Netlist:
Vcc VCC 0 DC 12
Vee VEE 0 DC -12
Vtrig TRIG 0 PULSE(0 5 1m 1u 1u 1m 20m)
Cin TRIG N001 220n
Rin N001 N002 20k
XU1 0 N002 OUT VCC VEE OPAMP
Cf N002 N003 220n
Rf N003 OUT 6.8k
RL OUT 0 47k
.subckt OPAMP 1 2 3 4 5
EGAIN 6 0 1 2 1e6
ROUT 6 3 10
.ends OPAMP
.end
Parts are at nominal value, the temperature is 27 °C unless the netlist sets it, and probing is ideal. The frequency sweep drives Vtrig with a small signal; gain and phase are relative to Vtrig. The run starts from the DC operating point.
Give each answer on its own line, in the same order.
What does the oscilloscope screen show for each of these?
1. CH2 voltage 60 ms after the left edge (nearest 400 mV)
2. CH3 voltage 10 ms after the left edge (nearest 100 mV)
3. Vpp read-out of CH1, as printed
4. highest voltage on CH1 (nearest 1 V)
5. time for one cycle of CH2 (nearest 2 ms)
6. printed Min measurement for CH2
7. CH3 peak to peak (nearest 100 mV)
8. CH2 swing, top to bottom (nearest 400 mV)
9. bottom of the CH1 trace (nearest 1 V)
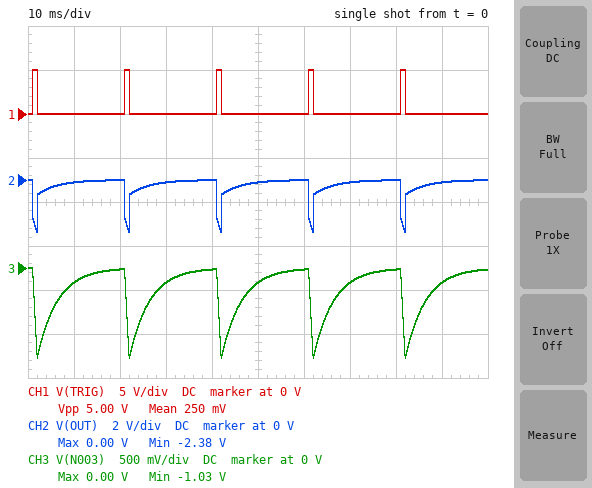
0 V
-200 mV
5.00 V
5 V
20 ms
-2.38 V
1.0 V
2.4 V
0 V
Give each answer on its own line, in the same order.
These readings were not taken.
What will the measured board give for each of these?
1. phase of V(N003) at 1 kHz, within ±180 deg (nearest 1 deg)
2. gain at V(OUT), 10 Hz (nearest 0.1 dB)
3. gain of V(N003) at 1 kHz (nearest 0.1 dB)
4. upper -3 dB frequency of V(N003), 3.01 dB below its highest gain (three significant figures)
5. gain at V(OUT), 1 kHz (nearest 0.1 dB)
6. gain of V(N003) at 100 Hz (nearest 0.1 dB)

92 deg
-0.3 dB
-28.8 dB
36.2 Hz
-9.3 dB
-9.4 dB
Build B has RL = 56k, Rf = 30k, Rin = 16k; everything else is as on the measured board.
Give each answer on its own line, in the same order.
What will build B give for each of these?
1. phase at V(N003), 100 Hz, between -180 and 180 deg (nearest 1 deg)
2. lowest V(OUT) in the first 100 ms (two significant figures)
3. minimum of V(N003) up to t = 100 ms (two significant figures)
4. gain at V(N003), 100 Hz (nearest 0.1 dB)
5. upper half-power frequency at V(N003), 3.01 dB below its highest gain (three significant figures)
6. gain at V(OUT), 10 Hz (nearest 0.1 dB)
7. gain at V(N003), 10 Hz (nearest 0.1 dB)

114 deg
-9.4 V
-1.2 V
-7.7 dB
45.2 Hz
0.5 dB
-0.2 dB
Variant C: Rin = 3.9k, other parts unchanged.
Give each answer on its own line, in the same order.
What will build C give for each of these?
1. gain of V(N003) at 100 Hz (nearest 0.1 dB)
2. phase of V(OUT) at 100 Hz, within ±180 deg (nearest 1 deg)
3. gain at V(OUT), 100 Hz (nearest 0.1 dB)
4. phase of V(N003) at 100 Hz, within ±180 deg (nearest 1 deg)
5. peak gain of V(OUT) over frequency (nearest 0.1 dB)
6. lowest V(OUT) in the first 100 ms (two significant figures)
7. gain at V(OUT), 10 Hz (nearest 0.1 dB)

-1.1 dB
-165 deg
1.6 dB
152 deg
4.8 dB
-8.7 V
0 dB
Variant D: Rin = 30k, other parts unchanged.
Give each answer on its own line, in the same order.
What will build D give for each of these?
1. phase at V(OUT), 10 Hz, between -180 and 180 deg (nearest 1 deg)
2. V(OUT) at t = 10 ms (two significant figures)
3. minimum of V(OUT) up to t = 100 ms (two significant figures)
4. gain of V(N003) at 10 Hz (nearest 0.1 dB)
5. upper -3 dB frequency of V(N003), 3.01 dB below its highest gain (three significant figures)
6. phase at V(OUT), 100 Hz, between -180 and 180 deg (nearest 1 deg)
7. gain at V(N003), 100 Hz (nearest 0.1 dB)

163 deg
-160 mV
-1.7 V
-0.7 dB
24.1 Hz
147 deg
-12.6 dB
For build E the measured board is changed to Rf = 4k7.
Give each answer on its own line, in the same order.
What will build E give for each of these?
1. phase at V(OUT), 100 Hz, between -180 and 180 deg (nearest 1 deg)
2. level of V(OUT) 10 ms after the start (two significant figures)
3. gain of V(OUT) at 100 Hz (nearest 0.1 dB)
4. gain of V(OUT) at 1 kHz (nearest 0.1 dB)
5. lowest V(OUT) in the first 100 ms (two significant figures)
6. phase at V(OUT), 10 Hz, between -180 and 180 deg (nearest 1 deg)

143 deg
-130 mV
-7.8 dB
-12.5 dB
-2.0 V
168 deg
